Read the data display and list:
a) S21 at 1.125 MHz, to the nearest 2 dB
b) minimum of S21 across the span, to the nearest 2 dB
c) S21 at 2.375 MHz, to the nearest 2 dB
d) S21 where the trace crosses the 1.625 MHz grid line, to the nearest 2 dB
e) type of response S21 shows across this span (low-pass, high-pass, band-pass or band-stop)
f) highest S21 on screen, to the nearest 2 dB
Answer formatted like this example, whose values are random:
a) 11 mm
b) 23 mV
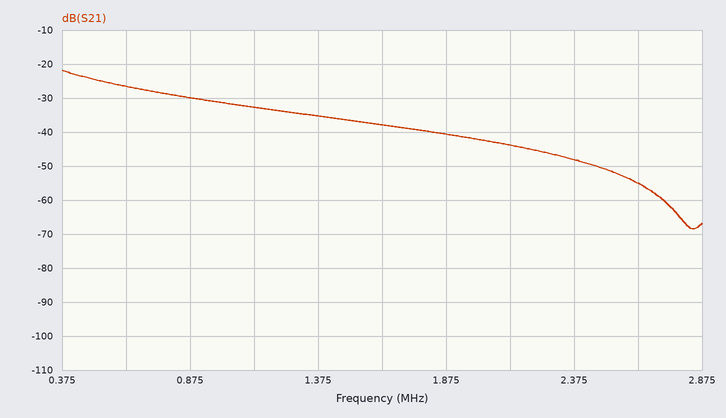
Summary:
a) -32 dB
b) -68 dB
c) -48 dB
d) -38 dB
e) low-pass
f) -22 dB
